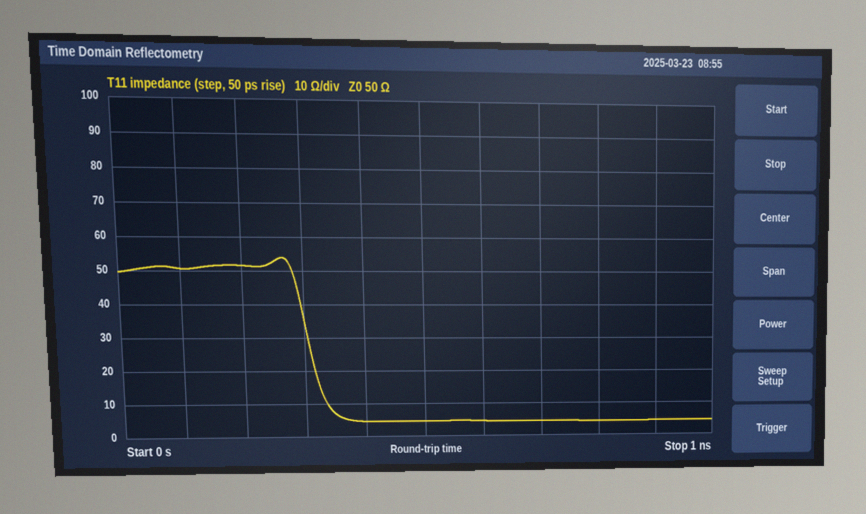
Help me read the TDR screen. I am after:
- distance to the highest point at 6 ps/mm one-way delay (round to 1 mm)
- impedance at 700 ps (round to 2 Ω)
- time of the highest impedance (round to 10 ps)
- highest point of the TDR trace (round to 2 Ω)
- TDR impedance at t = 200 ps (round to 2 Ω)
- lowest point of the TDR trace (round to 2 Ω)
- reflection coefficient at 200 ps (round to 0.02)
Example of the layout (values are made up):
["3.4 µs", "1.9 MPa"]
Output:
["22 mm", "4 Ω", "270 ps", "54 Ω", "52 Ω", "4 Ω", "+0.02"]
